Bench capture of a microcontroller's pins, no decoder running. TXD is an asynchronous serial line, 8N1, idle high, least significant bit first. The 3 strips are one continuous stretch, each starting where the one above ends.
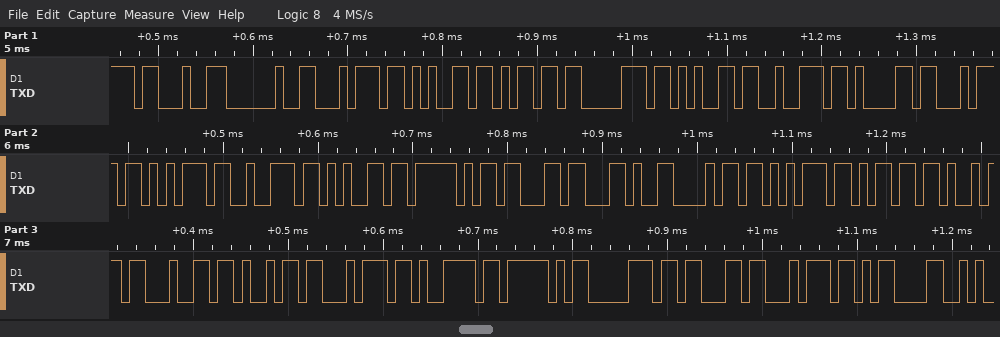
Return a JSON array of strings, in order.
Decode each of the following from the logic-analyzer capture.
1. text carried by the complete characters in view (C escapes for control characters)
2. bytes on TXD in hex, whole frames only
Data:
["\"# temperature_c,humidity_pct\\r\"", "23 20 74 65 6D 70 65 72 61 74 75 72 65 5F 63 2C 68 75 6D 69 64 69 74 79 5F 70 63 74 0D"]
